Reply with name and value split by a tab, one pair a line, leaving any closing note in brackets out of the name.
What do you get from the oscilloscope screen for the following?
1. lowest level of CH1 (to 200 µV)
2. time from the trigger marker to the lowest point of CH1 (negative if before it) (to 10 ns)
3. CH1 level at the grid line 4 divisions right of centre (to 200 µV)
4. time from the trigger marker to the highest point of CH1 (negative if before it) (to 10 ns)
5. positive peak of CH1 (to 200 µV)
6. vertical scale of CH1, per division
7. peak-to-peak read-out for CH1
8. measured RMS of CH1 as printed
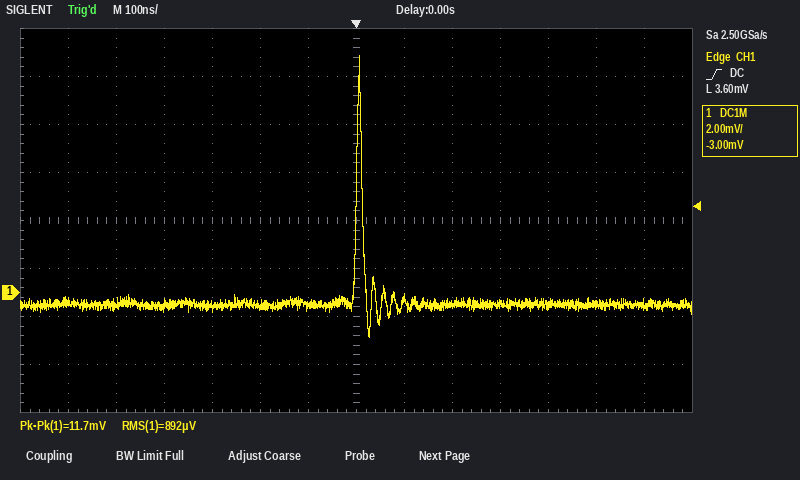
lowest level of CH1	-1.8 mV
time from the trigger marker to the lowest point of CH1 (negative if before it)	+30 ns
CH1 level at the grid line 4 divisions right of centre	-600 µV
time from the trigger marker to the highest point of CH1 (negative if before it)	+10 ns
positive peak of CH1	9.8 mV
vertical scale of CH1, per division	2 mV
peak-to-peak read-out for CH1	11.7 mV
measured RMS of CH1 as printed	892 µV
